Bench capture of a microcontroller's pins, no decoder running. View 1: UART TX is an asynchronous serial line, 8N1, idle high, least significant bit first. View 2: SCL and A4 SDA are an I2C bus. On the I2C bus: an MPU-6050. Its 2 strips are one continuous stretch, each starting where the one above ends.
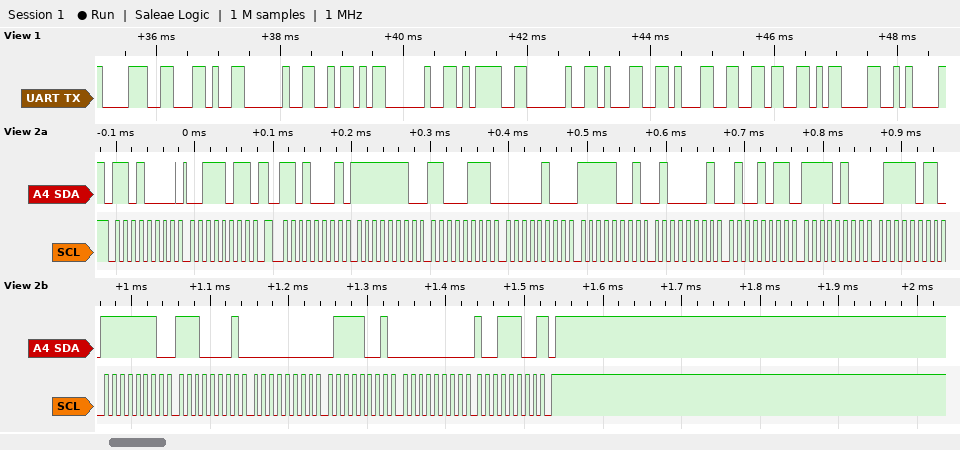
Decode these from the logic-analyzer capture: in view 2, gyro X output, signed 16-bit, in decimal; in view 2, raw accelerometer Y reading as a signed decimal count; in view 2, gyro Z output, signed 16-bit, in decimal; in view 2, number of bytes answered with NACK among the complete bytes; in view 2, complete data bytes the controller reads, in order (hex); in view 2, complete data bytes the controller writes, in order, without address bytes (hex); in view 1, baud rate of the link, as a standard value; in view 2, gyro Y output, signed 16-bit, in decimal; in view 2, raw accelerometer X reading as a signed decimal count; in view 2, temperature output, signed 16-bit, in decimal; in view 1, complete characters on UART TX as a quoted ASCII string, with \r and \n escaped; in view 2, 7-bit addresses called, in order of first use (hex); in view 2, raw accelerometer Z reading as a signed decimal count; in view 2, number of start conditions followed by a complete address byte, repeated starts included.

-287
1273
156
1
FE C7 04 F9 41 4B F4 7B FE E1 00 79 00 9C
3B
9600 baud
121
-313
-2949
"8, Z = 116\r\n"
0x68
16715
2
